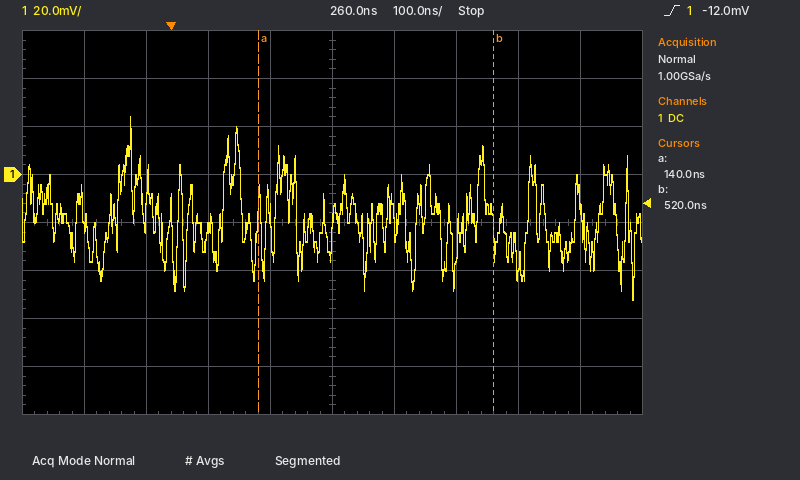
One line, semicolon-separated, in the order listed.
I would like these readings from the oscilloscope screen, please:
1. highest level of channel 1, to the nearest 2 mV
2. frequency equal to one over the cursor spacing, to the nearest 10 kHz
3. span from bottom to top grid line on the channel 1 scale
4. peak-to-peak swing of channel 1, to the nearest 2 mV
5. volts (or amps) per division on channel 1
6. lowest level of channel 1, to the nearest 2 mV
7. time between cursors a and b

24 mV; 2.63 MHz; 160 mV; 76 mV; 20 mV; -52 mV; 380 ns
